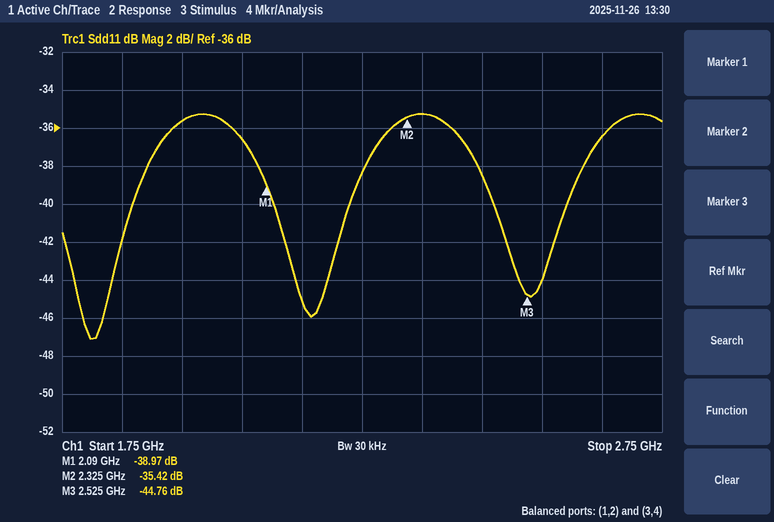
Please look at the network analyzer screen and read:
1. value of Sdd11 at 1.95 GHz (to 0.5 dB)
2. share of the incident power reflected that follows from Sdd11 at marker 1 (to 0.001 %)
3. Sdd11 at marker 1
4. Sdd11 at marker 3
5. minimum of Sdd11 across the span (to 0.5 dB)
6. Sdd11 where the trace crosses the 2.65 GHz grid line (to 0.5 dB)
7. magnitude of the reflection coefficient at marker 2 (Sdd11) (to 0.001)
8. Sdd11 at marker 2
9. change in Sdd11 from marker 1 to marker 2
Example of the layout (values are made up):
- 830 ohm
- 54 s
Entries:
- -35.5 dB
- 0.013 %
- -38.97 dB
- -44.76 dB
- -47.0 dB
- -36.5 dB
- 0.017
- -35.42 dB
- 3.55 dB
